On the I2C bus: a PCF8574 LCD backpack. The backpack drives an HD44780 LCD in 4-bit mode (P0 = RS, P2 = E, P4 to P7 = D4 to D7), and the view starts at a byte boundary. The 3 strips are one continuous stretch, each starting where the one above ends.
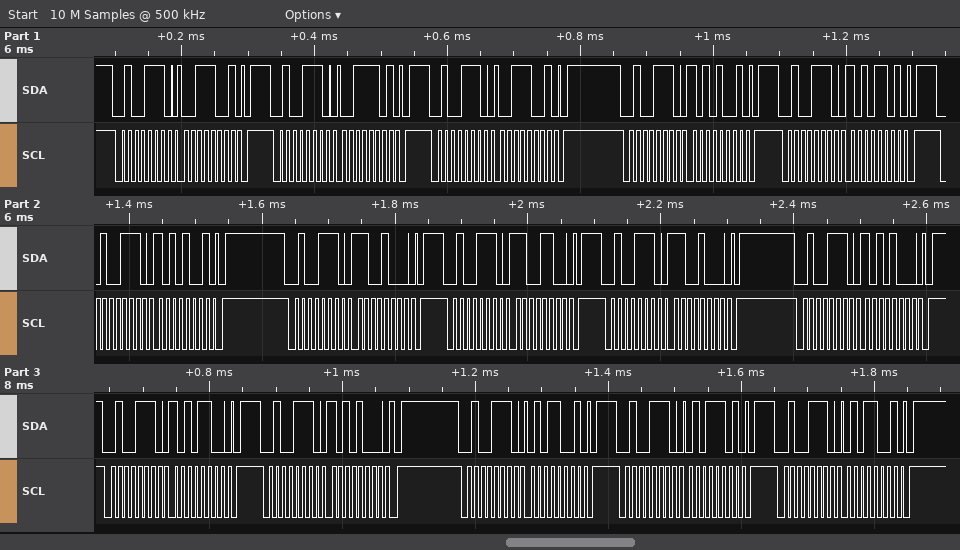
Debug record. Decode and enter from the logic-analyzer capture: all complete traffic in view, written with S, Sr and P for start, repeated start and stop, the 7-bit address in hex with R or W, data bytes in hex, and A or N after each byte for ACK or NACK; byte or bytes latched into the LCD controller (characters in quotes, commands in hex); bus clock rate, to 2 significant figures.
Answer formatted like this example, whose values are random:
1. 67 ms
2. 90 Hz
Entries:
1. S 27W A 39 A P S 27W A 3D A P S 27W A 39 A P S 27W A A9 A P S 27W A AD A P S 27W A A9 A P S 27W A C8 A P S 27W A CC A P S 27W A C8 A P S 27W A A8 A P S 27W A AC A P S 27W A A8 A P S 27W A 59 A P S 27W A 5D A P S 27W A 59 A P
2. ':' 0xCA
3. 100 kHz
